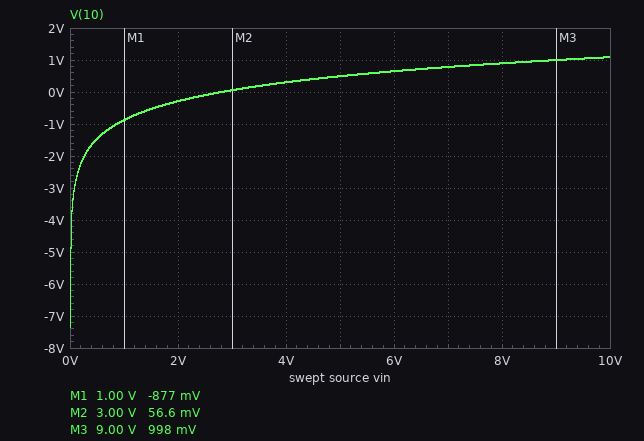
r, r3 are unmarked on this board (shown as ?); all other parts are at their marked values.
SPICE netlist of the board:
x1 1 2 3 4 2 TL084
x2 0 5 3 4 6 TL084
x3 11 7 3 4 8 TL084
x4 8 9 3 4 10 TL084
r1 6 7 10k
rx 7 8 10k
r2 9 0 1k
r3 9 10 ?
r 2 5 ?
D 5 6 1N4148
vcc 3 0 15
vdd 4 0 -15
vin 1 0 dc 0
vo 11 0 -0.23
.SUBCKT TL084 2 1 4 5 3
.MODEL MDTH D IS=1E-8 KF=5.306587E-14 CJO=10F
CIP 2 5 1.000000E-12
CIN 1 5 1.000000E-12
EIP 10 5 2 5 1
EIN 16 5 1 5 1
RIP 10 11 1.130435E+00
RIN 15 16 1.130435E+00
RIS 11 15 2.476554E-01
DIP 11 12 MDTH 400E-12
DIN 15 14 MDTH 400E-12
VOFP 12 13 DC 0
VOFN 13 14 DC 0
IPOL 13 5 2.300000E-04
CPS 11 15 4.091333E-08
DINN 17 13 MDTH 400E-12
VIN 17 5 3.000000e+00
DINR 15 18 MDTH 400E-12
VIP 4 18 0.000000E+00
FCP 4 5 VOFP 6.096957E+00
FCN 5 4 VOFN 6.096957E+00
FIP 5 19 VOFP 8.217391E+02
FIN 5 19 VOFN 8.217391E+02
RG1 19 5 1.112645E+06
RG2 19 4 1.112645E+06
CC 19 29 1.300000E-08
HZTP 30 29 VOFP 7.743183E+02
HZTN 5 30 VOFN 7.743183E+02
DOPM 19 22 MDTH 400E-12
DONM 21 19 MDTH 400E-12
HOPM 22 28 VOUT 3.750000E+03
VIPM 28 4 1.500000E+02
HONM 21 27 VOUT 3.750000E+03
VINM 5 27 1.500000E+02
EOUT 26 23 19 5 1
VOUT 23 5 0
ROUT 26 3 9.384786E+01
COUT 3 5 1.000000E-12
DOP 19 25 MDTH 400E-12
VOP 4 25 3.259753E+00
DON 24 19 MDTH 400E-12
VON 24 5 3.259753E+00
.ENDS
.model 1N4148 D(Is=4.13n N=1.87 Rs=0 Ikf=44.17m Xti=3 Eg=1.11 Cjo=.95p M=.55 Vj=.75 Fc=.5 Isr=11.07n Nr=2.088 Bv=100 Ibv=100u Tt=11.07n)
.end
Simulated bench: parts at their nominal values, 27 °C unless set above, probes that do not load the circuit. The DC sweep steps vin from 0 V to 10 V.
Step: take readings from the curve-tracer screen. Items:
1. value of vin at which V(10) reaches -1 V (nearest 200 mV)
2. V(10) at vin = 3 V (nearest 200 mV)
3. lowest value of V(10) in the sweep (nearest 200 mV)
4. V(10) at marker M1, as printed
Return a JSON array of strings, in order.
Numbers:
["800 mV", "0 V", "-7.4 V", "-877 mV"]
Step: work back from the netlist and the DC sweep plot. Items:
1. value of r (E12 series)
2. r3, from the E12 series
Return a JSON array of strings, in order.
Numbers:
["33 kΩ", "15 kΩ"]
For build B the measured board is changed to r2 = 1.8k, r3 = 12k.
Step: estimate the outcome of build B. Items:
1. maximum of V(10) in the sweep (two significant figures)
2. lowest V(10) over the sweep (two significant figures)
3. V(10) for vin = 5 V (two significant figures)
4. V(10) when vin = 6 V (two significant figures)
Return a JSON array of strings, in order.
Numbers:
["520 mV", "-3.5 V", "240 mV", "310 mV"]
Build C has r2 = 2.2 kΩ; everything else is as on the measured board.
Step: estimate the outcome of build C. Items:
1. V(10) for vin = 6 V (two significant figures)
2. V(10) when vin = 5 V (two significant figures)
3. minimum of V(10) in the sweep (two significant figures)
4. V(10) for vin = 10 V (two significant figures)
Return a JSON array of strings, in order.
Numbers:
["320 mV", "240 mV", "-3.6 V", "530 mV"]
